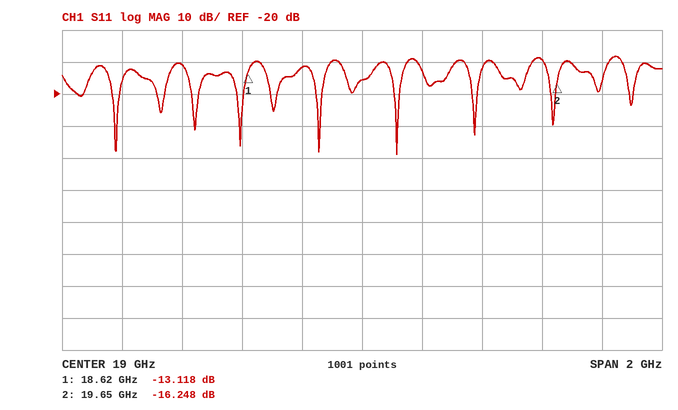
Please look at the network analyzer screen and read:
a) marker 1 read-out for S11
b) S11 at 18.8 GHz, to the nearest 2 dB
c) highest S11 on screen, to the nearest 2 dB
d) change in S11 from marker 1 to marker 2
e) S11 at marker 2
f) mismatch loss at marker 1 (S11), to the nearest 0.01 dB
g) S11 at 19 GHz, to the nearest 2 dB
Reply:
-13.118 dB
-12 dB
-8 dB
-3.130 dB
-16.248 dB
0.22 dB
-16 dB
